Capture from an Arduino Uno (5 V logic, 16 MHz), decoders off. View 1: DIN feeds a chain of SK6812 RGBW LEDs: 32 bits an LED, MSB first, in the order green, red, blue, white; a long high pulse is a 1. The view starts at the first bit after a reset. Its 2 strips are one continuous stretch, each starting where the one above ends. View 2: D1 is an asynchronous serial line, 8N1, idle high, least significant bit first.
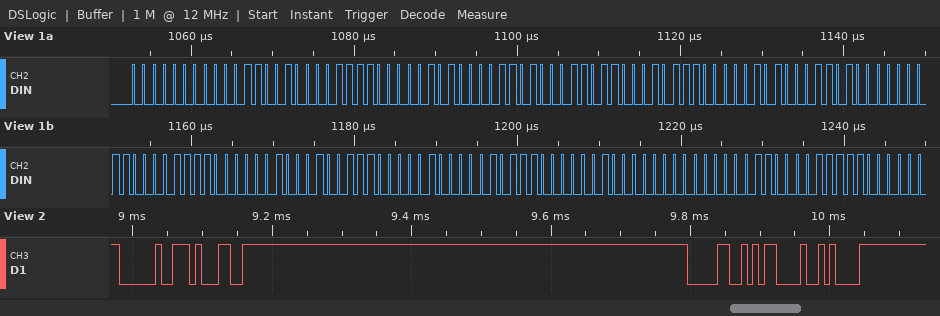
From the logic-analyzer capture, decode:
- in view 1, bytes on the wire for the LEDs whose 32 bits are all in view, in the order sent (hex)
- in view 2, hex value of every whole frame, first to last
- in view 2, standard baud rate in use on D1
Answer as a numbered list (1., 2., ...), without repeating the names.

1. 00 19 0F 05 0D 1B 17 05 1A 03 0F 02 27 04 17 02
2. 20 31 30 0D 0A
3. 115200 baud
